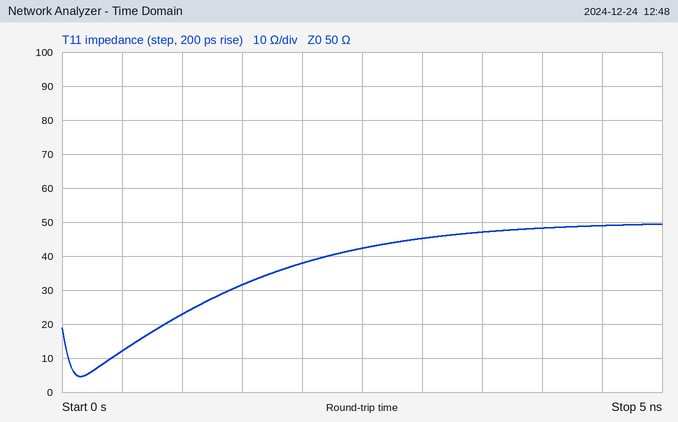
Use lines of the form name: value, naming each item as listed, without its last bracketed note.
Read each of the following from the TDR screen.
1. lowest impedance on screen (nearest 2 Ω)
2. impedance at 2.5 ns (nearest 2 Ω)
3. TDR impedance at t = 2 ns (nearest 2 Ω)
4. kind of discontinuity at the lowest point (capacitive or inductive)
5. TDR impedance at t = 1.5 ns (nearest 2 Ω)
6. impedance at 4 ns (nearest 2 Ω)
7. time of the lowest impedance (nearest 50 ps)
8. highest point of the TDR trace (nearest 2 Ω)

lowest impedance on screen: 4 Ω
impedance at 2.5 ns: 42 Ω
TDR impedance at t = 2 ns: 38 Ω
kind of discontinuity at the lowest point: capacitive
TDR impedance at t = 1.5 ns: 32 Ω
impedance at 4 ns: 48 Ω
time of the lowest impedance: 150 ps
highest point of the TDR trace: 50 Ω
